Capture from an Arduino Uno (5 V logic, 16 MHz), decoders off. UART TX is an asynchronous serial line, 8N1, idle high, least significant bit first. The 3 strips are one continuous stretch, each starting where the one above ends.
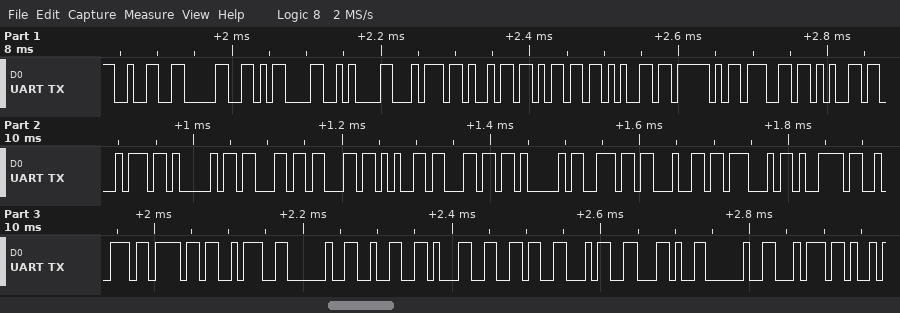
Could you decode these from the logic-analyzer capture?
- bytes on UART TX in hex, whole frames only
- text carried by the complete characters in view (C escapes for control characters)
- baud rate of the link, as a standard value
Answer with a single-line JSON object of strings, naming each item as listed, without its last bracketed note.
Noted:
{"bytes on UART TX in hex, whole frames only": "32 30 0D 0A 74 69 6D 65 5F 67 65 74 41 63 63 65 6C 41 6E 64 47 79 72 6F 3A 20 32 31 36 34 2C 20 74", "text carried by the complete characters in view": "\"20\\r\\ntime_getAccelAndGyro: 2164, t\"", "baud rate of the link, as a standard value": "115200 baud"}
